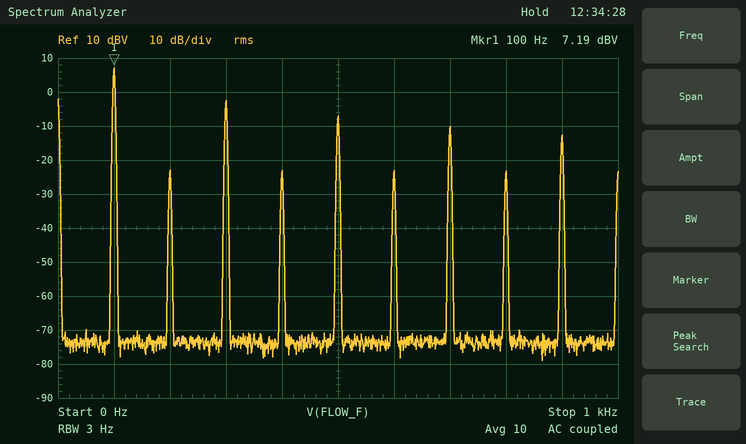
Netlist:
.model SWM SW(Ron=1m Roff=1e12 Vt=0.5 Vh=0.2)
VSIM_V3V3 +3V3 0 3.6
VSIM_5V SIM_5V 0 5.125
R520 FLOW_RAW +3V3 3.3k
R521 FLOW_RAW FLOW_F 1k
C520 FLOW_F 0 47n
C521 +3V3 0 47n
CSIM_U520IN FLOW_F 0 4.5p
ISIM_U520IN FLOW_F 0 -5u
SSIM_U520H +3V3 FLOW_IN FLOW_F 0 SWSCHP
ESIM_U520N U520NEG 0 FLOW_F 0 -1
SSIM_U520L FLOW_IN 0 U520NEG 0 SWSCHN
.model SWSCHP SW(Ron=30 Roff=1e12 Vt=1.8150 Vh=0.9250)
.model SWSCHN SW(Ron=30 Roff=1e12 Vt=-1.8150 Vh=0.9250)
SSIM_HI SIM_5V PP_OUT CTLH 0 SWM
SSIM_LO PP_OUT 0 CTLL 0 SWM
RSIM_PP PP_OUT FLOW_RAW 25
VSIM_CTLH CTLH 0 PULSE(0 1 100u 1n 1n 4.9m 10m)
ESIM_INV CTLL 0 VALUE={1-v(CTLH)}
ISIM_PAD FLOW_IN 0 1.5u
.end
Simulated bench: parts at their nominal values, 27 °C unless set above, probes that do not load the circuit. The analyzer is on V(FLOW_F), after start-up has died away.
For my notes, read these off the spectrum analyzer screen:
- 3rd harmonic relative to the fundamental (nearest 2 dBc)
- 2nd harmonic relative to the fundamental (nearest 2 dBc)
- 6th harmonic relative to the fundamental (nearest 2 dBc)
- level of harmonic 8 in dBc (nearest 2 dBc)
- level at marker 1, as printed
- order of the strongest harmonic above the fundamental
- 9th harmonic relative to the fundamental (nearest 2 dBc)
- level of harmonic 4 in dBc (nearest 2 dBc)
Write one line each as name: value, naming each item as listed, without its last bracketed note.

3rd harmonic relative to the fundamental: -10 dBc
2nd harmonic relative to the fundamental: -30 dBc
6th harmonic relative to the fundamental: -30 dBc
level of harmonic 8 in dBc: -30 dBc
level at marker 1, as printed: 7.19 dBV
order of the strongest harmonic above the fundamental: 3
9th harmonic relative to the fundamental: -20 dBc
level of harmonic 4 in dBc: -30 dBc
